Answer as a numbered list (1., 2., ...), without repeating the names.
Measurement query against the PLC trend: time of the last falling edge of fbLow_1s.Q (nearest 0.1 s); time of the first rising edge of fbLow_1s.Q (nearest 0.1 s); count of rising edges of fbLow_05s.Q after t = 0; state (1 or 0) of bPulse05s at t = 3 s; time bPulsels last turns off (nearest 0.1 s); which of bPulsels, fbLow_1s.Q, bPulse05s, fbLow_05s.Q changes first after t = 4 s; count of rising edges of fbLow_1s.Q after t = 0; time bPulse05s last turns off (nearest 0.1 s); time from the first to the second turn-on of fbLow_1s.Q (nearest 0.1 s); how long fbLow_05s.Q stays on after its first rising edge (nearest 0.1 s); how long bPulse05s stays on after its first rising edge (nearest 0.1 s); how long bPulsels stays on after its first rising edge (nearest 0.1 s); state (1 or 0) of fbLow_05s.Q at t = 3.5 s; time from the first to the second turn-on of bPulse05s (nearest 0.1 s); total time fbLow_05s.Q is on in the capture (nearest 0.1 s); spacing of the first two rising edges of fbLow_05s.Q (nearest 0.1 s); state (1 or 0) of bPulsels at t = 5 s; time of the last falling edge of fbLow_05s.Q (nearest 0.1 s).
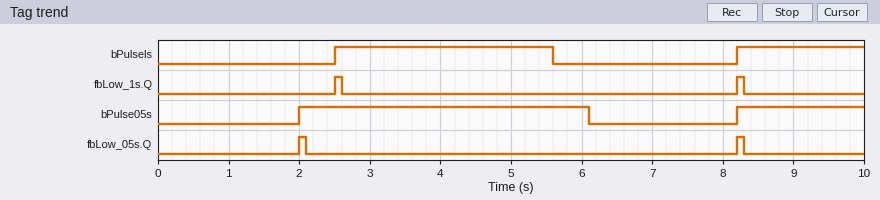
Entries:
1. 8.3 s
2. 2.5 s
3. 2
4. 1
5. 5.6 s
6. bPulsels
7. 2
8. 6.1 s
9. 5.7 s
10. 0.1 s
11. 4.1 s
12. 3.1 s
13. 0
14. 6.2 s
15. 0.2 s
16. 6.2 s
17. 1
18. 8.3 s
